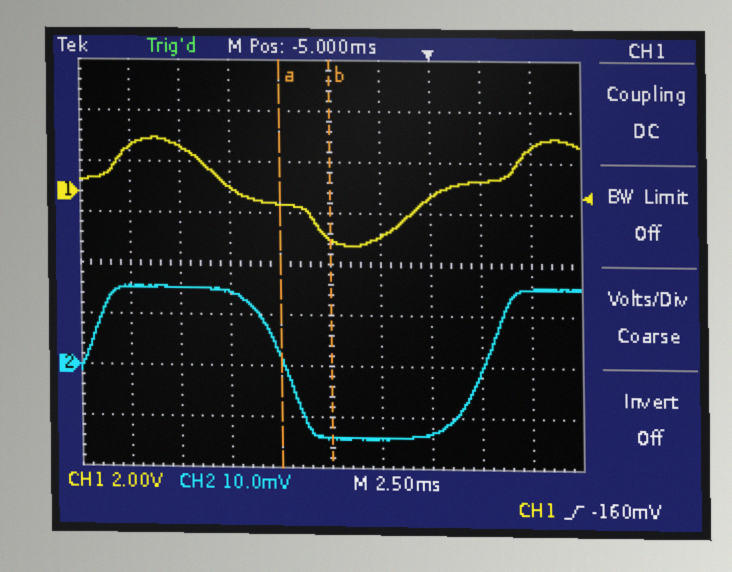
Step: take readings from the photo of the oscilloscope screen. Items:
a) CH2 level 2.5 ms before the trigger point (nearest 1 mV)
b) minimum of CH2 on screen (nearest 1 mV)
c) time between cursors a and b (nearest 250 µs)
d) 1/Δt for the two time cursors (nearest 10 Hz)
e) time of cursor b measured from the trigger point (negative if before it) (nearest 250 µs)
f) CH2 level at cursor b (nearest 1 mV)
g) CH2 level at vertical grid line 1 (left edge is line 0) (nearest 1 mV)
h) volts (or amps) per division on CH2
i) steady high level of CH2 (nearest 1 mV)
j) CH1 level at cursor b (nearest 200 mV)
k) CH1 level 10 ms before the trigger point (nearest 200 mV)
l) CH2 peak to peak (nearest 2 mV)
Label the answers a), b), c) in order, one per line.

a) -14 mV
b) -14 mV
c) 2.50 ms
d) 400 Hz
e) -5.00 ms
f) -14 mV
g) 15 mV
h) 10 mV
i) 15 mV
j) -1.8 V
k) 200 mV
l) 30 mV
